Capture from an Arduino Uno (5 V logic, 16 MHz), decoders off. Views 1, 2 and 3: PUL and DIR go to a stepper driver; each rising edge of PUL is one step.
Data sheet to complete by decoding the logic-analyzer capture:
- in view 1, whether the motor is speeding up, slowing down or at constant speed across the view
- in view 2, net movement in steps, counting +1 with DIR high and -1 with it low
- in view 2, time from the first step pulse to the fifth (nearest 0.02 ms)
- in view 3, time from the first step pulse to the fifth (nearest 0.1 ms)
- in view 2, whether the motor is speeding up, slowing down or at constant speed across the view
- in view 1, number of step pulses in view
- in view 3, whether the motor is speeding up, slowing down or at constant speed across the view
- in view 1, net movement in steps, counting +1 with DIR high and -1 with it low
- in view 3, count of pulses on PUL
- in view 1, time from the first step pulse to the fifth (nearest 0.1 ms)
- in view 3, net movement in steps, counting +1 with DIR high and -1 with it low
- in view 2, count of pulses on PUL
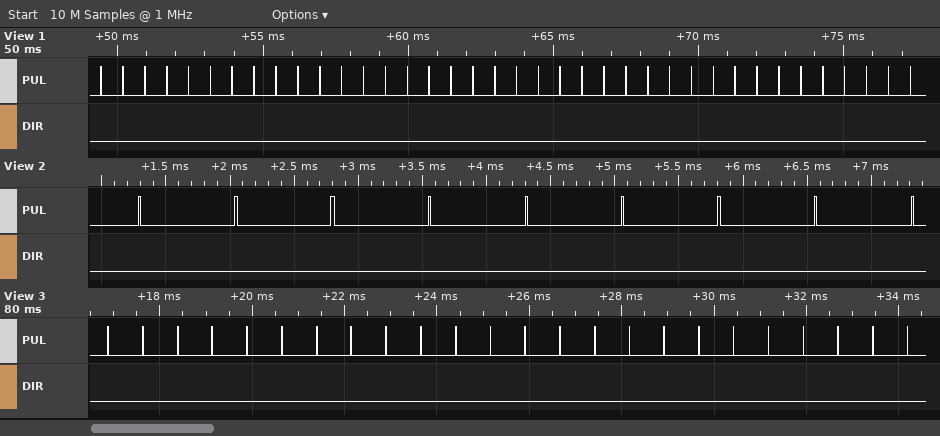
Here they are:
constant speed
-9
3.02 ms
3.0 ms
constant speed
38
constant speed
-38
24
3.0 ms
-24
9
